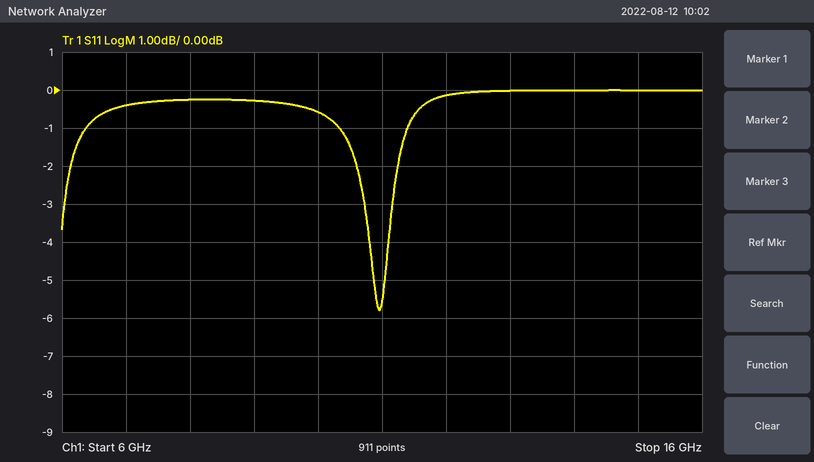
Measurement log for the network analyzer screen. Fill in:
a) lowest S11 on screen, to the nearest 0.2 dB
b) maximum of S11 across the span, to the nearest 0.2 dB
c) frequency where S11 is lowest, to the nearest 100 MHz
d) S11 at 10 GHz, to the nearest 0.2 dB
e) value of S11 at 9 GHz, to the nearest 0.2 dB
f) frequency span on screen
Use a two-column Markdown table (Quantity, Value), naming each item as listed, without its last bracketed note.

| Quantity | Value |
|---|---|
| lowest S11 on screen, to the nearest 0.2 dB | -5.8 dB |
| maximum of S11 across the span, to the nearest 0.2 dB | 0.0 dB |
| frequency where S11 is lowest, to the nearest 100 MHz | 11.0 GHz |
| S11 at 10 GHz, to the nearest 0.2 dB | -0.6 dB |
| value of S11 at 9 GHz, to the nearest 0.2 dB | -0.2 dB |
| frequency span on screen | 10 GHz |
